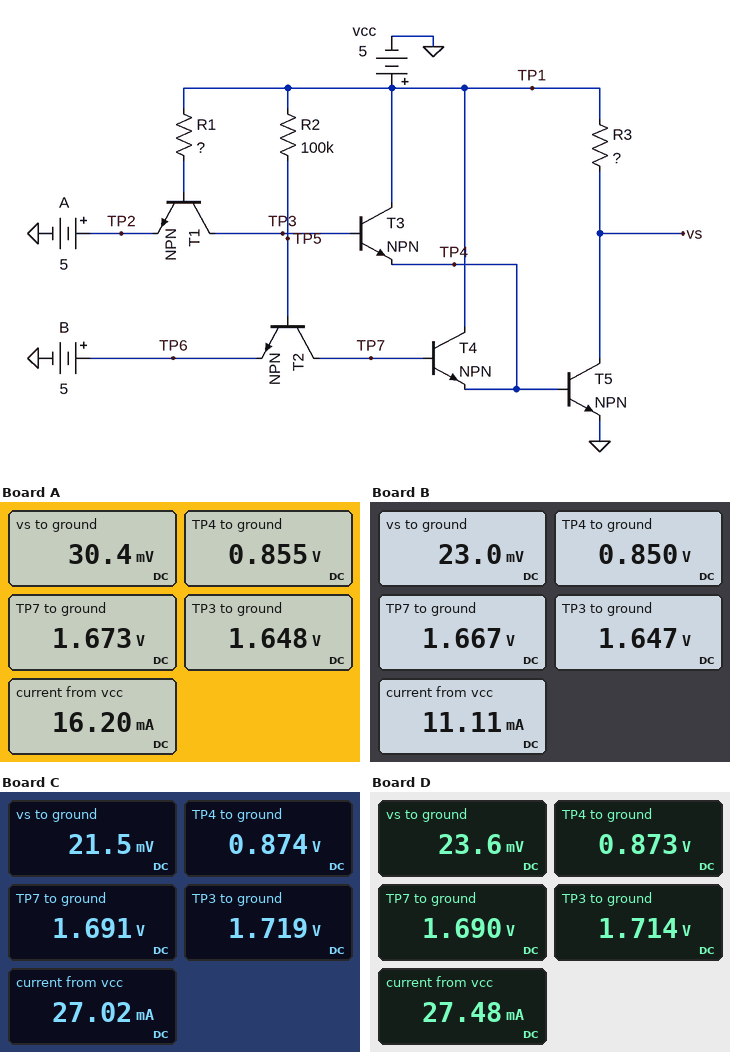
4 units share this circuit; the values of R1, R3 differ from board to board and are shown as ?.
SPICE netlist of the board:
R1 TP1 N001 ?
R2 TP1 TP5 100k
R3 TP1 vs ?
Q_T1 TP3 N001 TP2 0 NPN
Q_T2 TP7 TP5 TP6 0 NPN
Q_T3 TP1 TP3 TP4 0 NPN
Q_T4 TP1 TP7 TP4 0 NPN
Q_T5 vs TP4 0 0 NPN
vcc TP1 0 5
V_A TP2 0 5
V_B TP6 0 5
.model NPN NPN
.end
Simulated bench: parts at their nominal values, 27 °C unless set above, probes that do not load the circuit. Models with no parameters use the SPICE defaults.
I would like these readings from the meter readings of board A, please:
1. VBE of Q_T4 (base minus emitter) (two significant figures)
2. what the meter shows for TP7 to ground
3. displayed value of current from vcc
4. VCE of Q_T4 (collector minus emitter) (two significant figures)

820 mV
1.673 V
16.20 mA
4.1 V
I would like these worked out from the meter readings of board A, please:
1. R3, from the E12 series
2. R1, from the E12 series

560 Ω
270 kΩ
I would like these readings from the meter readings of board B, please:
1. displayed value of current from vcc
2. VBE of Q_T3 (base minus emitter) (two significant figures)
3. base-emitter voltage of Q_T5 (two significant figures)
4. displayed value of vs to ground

11.11 mA
800 mV
850 mV
23.0 mV
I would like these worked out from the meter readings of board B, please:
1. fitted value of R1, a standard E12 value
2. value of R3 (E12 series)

220 kΩ
1.5 kΩ
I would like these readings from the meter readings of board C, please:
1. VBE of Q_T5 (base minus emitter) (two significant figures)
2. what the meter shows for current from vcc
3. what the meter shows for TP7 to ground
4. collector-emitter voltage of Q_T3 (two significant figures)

870 mV
27.02 mA
1.691 V
4.1 V
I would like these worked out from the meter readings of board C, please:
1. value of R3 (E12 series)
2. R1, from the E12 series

820 Ω
33 kΩ
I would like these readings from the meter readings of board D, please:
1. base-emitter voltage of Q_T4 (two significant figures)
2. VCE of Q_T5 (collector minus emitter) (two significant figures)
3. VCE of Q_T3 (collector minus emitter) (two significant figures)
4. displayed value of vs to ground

820 mV
24 mV
4.1 V
23.6 mV
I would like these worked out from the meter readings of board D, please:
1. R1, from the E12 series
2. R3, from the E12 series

39 kΩ
560 Ω
